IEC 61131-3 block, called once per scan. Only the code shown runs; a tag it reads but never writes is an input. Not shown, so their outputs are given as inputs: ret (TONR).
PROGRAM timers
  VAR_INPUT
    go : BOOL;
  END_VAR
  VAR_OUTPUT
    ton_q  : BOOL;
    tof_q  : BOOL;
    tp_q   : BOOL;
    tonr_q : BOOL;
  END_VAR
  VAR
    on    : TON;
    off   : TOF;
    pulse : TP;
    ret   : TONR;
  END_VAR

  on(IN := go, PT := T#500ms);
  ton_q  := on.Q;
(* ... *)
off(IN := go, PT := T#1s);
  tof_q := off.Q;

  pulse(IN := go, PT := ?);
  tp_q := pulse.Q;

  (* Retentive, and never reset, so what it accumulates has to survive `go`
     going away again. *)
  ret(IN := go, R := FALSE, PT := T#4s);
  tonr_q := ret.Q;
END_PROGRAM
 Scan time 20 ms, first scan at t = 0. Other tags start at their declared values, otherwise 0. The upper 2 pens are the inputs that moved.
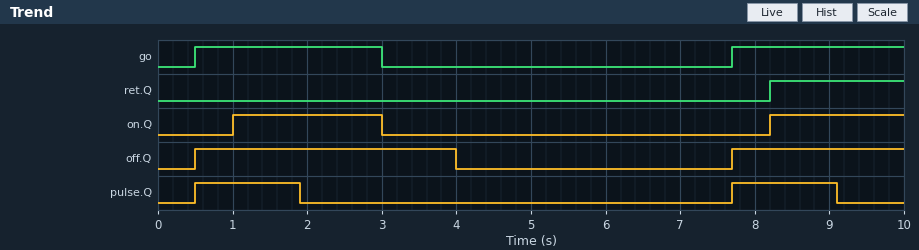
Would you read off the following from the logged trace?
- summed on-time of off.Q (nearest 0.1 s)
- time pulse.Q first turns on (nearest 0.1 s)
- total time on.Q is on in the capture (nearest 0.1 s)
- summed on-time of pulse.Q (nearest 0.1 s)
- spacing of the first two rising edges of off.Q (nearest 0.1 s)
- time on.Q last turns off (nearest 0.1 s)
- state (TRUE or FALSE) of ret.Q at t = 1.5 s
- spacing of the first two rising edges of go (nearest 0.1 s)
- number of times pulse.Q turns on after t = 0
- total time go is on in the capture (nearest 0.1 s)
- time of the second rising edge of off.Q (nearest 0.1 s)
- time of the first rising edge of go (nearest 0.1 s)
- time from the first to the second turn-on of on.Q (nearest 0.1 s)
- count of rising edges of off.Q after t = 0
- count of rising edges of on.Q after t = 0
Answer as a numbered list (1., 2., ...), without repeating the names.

1. 5.8 s
2. 0.5 s
3. 3.8 s
4. 2.8 s
5. 7.2 s
6. 3.0 s
7. FALSE
8. 7.2 s
9. 2
10. 4.8 s
11. 7.7 s
12. 0.5 s
13. 7.2 s
14. 2
15. 2
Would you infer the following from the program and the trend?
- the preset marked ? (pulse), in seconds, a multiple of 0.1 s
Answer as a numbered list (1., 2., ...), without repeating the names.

1. 1.4 s
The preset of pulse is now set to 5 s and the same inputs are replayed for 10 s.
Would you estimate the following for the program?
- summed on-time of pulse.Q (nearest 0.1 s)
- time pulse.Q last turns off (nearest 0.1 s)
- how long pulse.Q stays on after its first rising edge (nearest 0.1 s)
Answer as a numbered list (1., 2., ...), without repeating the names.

1. 7.3 s
2. 5.5 s
3. 5.0 s
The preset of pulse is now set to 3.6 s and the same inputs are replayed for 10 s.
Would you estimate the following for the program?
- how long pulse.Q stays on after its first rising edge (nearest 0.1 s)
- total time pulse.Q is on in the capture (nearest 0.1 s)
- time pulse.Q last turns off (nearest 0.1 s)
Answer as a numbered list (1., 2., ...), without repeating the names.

1. 3.6 s
2. 5.9 s
3. 4.1 s
